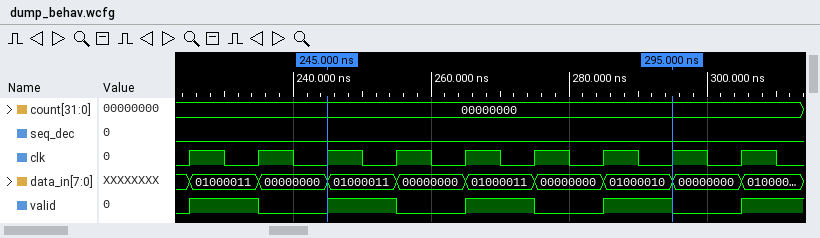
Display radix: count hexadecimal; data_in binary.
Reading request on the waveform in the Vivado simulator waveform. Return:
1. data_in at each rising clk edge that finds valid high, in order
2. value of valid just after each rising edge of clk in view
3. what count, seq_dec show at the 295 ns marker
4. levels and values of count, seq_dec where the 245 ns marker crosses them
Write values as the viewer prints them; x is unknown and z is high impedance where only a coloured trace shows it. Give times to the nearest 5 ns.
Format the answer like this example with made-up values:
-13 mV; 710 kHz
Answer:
01000011, 01000011, 01000011, 01000010; 1 0 1 0 1 0 1 0 1; count=00000000, seq_dec=0; count=00000000, seq_dec=0
